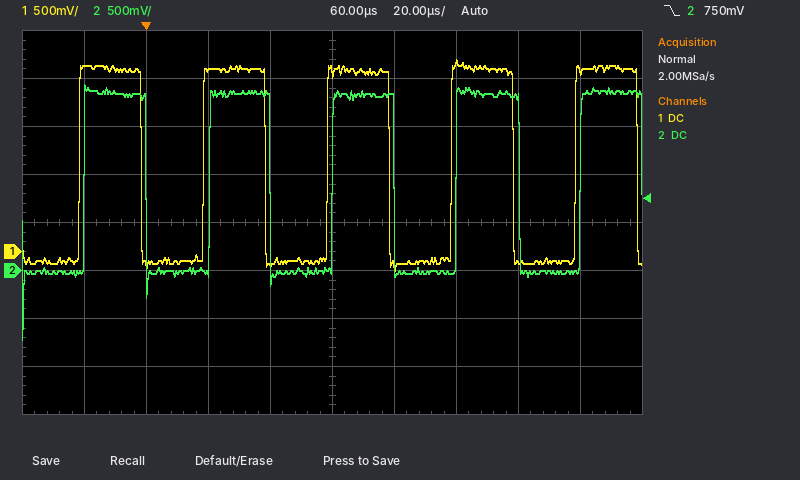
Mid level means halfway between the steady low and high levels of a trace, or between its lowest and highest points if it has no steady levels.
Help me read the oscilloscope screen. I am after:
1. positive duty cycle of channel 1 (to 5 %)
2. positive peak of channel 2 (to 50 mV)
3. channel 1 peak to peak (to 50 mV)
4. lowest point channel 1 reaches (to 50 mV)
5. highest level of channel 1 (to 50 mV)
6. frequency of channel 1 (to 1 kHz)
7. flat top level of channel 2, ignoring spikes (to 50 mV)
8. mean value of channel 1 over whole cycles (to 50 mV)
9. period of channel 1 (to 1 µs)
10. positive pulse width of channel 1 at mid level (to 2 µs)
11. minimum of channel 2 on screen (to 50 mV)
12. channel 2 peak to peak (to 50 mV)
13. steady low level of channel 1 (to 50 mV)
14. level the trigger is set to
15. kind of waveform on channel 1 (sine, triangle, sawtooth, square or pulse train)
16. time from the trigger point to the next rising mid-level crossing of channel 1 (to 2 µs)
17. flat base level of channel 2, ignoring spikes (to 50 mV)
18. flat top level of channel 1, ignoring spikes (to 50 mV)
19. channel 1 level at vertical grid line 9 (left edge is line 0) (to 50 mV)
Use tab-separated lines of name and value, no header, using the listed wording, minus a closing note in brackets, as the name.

positive duty cycle of channel 1	50 %
positive peak of channel 2	1.95 V
channel 1 peak to peak	2.20 V
lowest point channel 1 reaches	-200 mV
highest level of channel 1	2.00 V
frequency of channel 1	25 kHz
flat top level of channel 2, ignoring spikes	1.85 V
mean value of channel 1 over whole cycles	900 mV
period of channel 1	40 µs
positive pulse width of channel 1 at mid level	20 µs
minimum of channel 2 on screen	-700 mV
channel 2 peak to peak	2.65 V
steady low level of channel 1	-100 mV
level the trigger is set to	750 mV
kind of waveform on channel 1	square
time from the trigger point to the next rising mid-level crossing of channel 1	18 µs
flat base level of channel 2, ignoring spikes	0 mV
flat top level of channel 1, ignoring spikes	1.90 V
channel 1 level at vertical grid line 9 (left edge is line 0)	1.90 V
